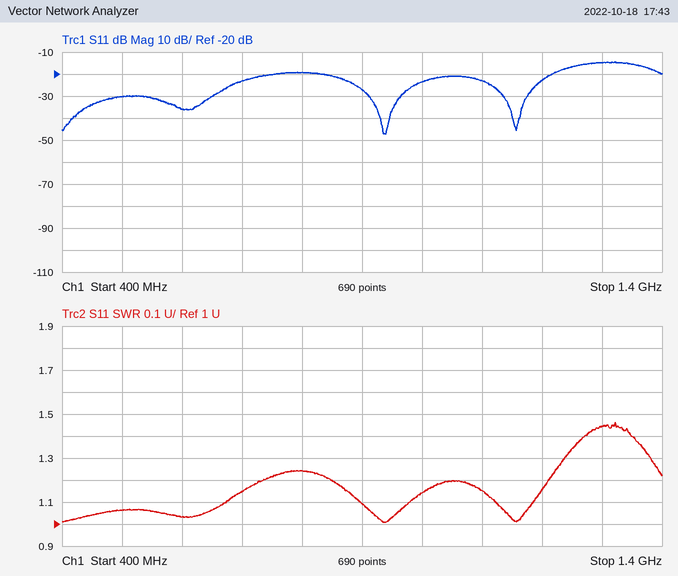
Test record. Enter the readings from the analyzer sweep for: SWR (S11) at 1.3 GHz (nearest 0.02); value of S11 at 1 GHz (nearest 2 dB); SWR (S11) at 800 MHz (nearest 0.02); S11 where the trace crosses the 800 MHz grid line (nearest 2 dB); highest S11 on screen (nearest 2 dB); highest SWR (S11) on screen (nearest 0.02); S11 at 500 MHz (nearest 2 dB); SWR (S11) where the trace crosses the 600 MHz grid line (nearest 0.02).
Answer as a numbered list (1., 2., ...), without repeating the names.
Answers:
1. 1.44
2. -24 dB
3. 1.24
4. -20 dB
5. -14 dB
6. 1.46
7. -30 dB
8. 1.04
